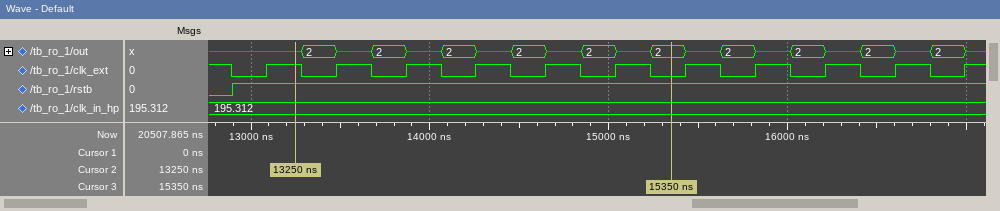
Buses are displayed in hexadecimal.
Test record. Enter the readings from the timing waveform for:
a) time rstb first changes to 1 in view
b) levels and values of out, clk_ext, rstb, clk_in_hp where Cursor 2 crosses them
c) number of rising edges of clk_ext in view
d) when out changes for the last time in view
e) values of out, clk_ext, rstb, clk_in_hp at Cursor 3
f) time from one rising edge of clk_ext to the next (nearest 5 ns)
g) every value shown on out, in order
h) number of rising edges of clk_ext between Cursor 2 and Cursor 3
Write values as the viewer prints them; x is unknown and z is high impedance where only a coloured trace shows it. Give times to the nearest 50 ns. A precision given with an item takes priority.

12900 ns
out=z, clk_ext=1, rstb=1, clk_in_hp=195.312
11
17000 ns
out=2, clk_ext=0, rstb=1, clk_in_hp=195.312
390 ns
z, 2, z, 2, z, 2, z, 2, z, 2, z, 2, z, 2, z, 2, z, 2, z, 2, z
5
